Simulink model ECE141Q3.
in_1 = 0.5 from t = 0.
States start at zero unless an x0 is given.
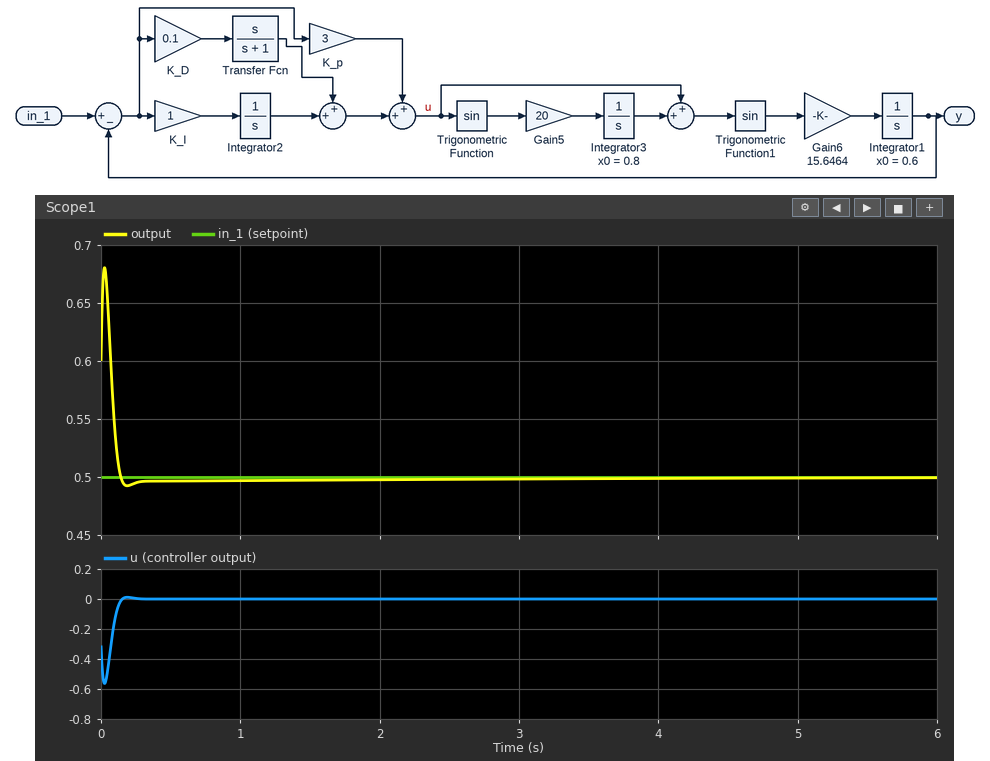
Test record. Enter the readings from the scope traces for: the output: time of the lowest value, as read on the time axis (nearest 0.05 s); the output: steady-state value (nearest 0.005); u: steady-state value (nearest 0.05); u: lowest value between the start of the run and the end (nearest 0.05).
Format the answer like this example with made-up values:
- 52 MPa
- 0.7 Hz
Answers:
- 0.20 s
- 0.500
- 0.00
- -0.55
